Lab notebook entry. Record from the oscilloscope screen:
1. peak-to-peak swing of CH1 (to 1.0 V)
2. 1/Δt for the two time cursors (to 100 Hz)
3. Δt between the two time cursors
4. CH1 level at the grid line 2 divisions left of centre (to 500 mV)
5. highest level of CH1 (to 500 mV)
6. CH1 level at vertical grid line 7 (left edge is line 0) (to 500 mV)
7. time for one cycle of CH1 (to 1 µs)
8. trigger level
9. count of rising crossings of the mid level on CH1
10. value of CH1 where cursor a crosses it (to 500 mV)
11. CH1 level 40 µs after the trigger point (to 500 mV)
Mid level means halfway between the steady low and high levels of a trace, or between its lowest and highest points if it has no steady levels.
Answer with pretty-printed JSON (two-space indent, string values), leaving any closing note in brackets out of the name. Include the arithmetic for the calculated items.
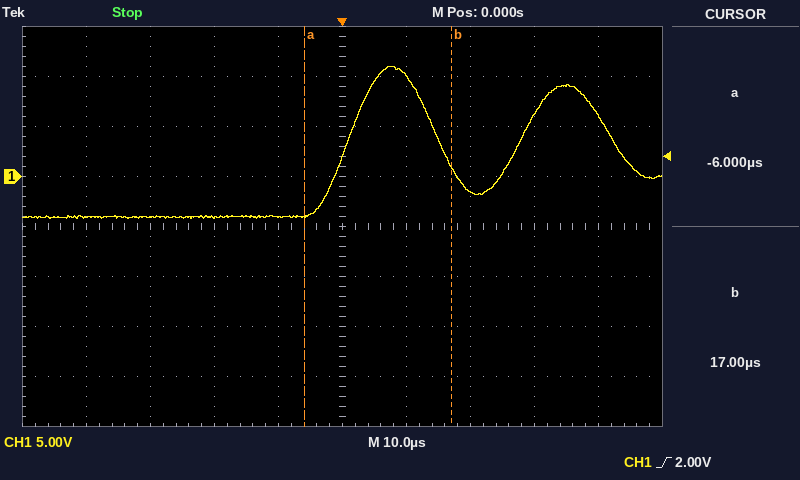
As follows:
{
  "peak-to-peak swing of CH1": "15.0 V",
  "1/Δt for the two time cursors": "1 / 23 µs ≈ 43.5 kHz",
  "Δt between the two time cursors": "17 µs − (-6 µs) = 23 µs",
  "CH1 level at the grid line 2 divisions left of centre": "-4.0 V",
  "highest level of CH1": "11.0 V",
  "CH1 level at vertical grid line 7 (left edge is line 0)": "-1.5 V",
  "time for one cycle of CH1": "27 µs",
  "trigger level": "2.00 V",
  "count of rising crossings of the mid level on CH1": "2",
  "value of CH1 where cursor a crosses it": "-4.0 V",
  "CH1 level 40 µs after the trigger point": "6.0 V"
}
